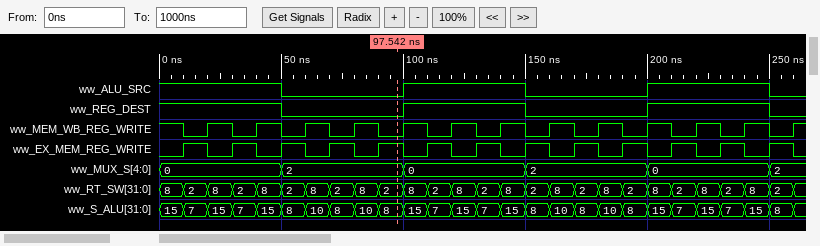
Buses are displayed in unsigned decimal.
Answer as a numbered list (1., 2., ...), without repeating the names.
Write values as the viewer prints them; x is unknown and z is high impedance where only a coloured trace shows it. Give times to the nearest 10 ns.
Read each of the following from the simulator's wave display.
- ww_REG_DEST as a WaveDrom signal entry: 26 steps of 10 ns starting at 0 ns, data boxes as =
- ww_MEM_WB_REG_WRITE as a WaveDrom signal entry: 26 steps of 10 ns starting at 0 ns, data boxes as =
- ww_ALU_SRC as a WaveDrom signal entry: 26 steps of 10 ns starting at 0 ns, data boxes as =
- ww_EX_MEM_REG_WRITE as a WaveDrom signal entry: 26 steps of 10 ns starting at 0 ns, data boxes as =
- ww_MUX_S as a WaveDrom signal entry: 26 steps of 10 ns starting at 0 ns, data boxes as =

1. {name: 'ww_REG_DEST', wave: '1....0....1....0....1....0'}
2. {name: 'ww_MEM_WB_REG_WRITE', wave: '10101010101010101010101010'}
3. {name: 'ww_ALU_SRC', wave: '1....0....1....0....1....0'}
4. {name: 'ww_EX_MEM_REG_WRITE', wave: '01010101010101010101010101'}
5. {name: 'ww_MUX_S', wave: '=....=....=....=....=....=', data: '0 2 0 2 0 2'}
